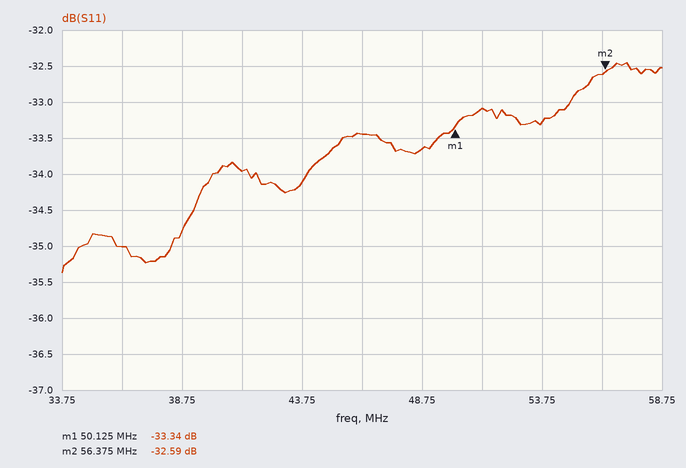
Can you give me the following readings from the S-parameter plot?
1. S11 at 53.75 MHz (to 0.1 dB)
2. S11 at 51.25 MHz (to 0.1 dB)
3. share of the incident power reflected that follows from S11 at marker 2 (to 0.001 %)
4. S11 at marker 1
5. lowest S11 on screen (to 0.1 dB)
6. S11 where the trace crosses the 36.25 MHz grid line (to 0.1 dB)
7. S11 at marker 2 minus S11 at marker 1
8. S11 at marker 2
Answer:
-33.3 dB
-33.1 dB
0.055 %
-33.34 dB
-35.4 dB
-35.0 dB
0.75 dB
-32.59 dB
